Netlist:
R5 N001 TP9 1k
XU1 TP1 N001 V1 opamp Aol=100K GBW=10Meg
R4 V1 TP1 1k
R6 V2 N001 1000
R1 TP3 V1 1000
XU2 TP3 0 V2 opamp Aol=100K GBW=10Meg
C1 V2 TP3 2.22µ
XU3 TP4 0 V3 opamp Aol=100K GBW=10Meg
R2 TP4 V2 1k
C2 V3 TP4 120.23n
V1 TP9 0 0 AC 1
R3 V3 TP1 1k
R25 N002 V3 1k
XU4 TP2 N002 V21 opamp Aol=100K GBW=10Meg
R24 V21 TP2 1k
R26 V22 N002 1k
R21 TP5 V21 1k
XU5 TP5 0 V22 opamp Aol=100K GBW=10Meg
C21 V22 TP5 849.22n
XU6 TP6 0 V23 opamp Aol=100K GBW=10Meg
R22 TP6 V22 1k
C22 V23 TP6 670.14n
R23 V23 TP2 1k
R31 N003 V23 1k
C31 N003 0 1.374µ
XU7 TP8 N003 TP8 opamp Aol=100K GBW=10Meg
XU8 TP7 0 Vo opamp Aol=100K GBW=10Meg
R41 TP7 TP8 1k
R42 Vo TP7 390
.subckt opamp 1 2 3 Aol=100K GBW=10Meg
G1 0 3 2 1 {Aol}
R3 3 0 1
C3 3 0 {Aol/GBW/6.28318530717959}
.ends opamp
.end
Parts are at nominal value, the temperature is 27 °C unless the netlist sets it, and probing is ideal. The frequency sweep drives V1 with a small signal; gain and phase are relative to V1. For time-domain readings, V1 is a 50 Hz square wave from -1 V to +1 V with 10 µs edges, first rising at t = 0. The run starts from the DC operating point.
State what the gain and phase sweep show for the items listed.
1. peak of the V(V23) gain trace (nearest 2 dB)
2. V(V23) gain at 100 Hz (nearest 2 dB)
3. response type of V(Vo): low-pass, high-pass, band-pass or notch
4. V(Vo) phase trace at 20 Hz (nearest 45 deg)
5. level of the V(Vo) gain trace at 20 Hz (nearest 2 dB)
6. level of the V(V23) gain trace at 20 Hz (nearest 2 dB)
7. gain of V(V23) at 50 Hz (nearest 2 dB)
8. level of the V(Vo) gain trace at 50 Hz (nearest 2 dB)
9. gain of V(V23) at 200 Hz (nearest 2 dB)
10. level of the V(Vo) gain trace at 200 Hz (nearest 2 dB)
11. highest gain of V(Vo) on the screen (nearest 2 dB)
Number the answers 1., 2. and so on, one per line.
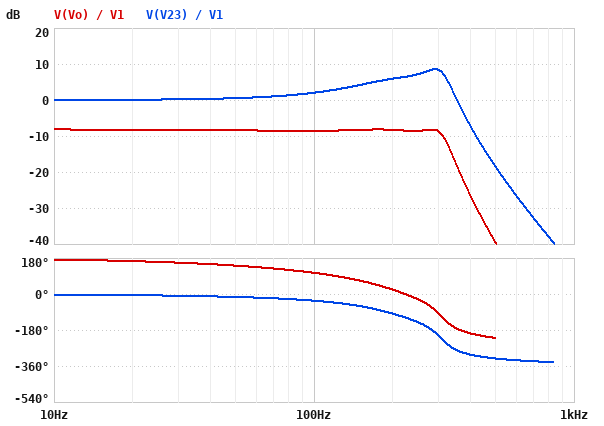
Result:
1. 8 dB
2. 2 dB
3. low-pass
4. 180 deg
5. -8 dB
6. 0 dB
7. 0 dB
8. -8 dB
9. 6 dB
10. -8 dB
11. -8 dB
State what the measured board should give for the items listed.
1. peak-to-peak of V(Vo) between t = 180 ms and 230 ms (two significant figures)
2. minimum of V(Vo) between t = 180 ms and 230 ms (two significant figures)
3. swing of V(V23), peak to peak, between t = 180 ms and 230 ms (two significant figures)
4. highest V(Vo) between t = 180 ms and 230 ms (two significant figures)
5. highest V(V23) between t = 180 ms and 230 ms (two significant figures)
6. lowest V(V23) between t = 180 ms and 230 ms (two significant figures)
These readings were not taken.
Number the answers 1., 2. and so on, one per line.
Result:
1. 980 mV
2. -490 mV
3. 4.4 V
4. 490 mV
5. 2.2 V
6. -2.2 V
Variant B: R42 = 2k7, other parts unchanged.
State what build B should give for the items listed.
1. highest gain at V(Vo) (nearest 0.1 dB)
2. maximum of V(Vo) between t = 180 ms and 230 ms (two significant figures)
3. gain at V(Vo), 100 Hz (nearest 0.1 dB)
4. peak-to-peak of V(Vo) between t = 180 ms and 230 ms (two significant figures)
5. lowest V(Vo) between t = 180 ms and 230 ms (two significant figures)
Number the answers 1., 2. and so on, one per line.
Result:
1. 8.6 dB
2. 3.4 V
3. 8.2 dB
4. 6.8 V
5. -3.4 V
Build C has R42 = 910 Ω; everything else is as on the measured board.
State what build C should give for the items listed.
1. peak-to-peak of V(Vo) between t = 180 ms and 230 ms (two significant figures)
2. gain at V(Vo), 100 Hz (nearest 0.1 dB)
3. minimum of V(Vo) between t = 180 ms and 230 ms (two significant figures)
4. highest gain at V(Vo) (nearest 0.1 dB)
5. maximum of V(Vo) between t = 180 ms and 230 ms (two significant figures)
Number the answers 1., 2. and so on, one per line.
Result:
1. 2.3 V
2. -1.2 dB
3. -1.1 V
4. -0.8 dB
5. 1.1 V
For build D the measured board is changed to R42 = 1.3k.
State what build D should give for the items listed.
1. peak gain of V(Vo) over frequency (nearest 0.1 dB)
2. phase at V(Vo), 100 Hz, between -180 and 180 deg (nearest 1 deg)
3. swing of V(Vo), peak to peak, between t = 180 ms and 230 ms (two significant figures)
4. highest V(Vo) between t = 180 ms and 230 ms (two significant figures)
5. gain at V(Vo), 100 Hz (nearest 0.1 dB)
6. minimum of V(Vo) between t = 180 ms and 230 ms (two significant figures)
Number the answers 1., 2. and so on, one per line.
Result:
1. 2.3 dB
2. 106 deg
3. 3.3 V
4. 1.6 V
5. 1.9 dB
6. -1.6 V
